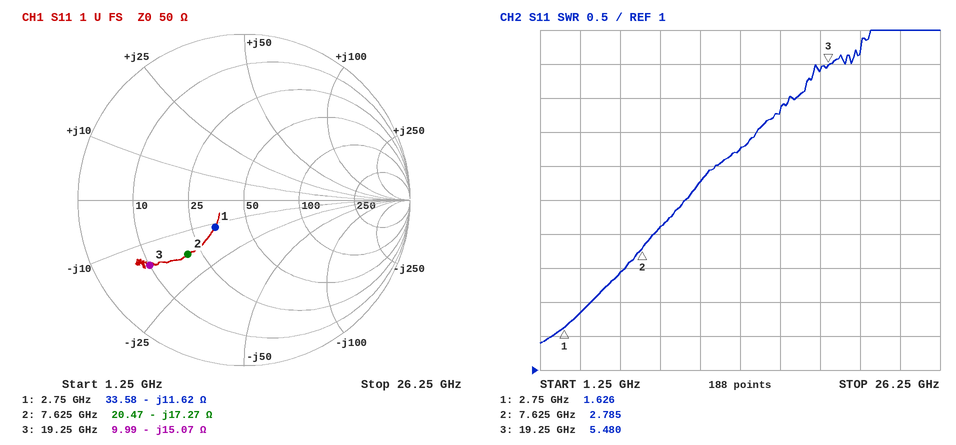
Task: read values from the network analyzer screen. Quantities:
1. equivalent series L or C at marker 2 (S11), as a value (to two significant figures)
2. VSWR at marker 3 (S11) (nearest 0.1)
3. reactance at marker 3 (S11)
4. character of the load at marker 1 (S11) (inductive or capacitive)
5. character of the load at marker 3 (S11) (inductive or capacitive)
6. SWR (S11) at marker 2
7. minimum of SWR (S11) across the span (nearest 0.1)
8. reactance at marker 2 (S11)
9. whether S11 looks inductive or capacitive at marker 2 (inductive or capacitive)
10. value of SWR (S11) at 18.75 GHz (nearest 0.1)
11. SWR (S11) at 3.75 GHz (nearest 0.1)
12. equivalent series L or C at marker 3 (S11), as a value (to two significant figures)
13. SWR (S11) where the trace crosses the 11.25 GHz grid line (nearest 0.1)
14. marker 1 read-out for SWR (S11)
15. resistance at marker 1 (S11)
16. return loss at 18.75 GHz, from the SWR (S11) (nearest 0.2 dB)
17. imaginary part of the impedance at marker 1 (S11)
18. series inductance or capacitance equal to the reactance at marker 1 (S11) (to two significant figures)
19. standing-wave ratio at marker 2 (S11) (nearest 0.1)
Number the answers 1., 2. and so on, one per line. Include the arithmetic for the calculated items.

1. C = 1/(2π × 7.625 GHz × 17.27 Ω) ≈ 1.2 pF
2. 5.5
3. -15.07 Ω
4. capacitive
5. capacitive
6. 2.785
7. 1.4
8. -17.27 Ω
9. capacitive
10. 5.4
11. 1.8
12. C = 1/(2π × 19.25 GHz × 15.07 Ω) ≈ 549 fF, so 550 fF to two significant figures
13. 3.8
14. 1.626
15. 33.58 Ω
16. −20 log10((5.4 − 1)/(5.4 + 1)) ≈ 3.2 dB
17. -11.62 Ω
18. C = 1/(2π × 2.75 GHz × 11.62 Ω) ≈ 5.0 pF
19. 2.8
